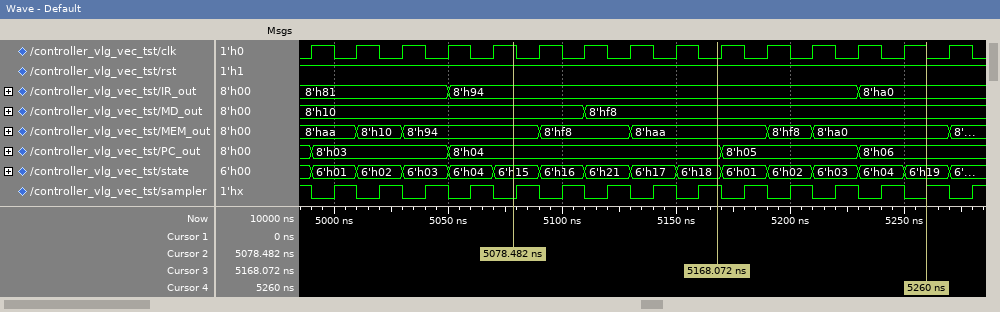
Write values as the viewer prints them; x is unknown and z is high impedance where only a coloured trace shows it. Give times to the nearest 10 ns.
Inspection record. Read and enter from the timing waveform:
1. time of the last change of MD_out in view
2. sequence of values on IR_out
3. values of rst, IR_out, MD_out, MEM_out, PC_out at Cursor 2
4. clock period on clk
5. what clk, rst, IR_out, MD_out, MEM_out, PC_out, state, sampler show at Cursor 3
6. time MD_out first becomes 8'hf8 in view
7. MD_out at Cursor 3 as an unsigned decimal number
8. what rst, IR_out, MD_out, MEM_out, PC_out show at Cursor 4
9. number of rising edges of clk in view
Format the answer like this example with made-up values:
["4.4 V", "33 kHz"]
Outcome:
["5110 ns", "8'h81, 8'h94, 8'ha0", "rst=1, IR_out=8'h94, MD_out=8'h10, MEM_out=8'h94, PC_out=8'h04", "20 ns", "clk=0, rst=1, IR_out=8'h94, MD_out=8'hf8, MEM_out=8'haa, PC_out=8'h04, state=6'h18, sampler=1", "5110 ns", "248", "rst=1, IR_out=8'ha0, MD_out=8'hf8, MEM_out=8'ha0, PC_out=8'h06", "15"]
